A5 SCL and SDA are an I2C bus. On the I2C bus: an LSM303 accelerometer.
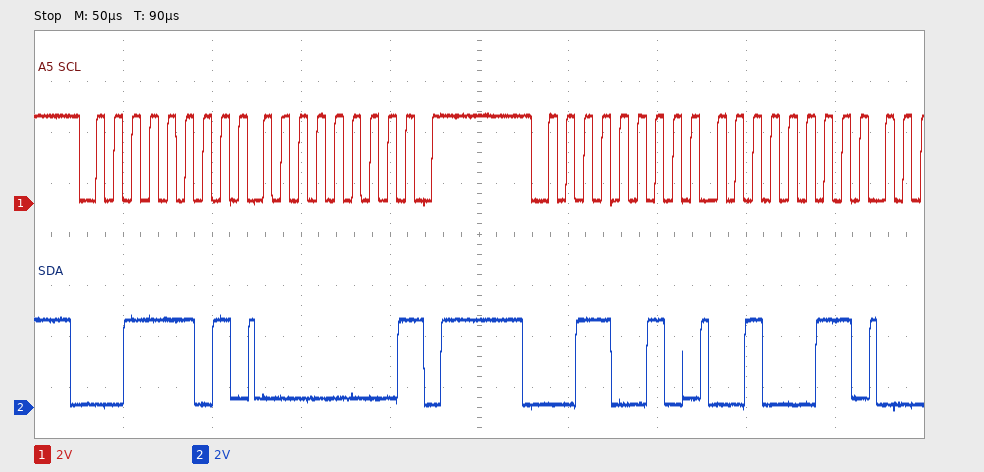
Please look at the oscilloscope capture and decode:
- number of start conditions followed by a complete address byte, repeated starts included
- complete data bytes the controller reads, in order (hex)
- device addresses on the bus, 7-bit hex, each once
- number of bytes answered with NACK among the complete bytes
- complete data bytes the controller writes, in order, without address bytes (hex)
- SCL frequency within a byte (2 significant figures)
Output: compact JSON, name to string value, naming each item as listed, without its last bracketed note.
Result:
{"number of start conditions followed by a complete address byte, repeated starts included": "2", "complete data bytes the controller reads, in order": "00", "device addresses on the bus, 7-bit hex, each once": "0x1E 0x19", "number of bytes answered with NACK among the complete bytes": "1", "complete data bytes the controller writes, in order, without address bytes": "23", "SCL frequency within a byte": "100 kHz"}
